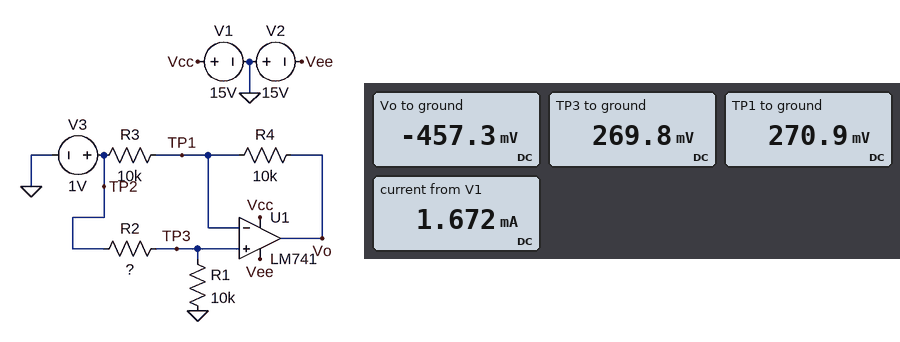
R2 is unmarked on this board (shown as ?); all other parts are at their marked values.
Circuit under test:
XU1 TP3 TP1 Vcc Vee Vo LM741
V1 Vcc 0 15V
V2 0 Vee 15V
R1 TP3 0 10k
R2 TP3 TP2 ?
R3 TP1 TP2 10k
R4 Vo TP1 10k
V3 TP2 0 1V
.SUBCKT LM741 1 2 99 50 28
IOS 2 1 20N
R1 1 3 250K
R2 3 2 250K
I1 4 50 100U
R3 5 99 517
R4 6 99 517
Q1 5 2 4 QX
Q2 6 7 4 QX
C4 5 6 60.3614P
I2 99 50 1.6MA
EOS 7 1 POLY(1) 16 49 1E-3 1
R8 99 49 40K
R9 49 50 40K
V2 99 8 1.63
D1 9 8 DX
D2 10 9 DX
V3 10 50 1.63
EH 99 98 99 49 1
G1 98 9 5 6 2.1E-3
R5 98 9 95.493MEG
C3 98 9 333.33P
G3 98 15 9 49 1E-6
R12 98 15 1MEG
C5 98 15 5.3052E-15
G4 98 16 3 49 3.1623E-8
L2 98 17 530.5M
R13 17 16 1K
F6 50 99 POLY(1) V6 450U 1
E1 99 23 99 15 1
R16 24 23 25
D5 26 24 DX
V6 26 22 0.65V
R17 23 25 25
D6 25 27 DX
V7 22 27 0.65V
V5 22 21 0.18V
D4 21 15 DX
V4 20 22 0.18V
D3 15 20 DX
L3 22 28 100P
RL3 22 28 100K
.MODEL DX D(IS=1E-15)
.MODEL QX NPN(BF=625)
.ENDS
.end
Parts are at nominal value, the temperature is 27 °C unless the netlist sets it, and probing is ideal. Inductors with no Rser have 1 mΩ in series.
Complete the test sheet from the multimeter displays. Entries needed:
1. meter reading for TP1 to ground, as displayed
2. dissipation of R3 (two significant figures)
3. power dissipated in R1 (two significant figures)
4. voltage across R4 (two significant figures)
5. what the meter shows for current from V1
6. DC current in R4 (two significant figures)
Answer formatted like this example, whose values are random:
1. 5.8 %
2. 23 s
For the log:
1. 270.9 mV
2. 53 µW
3. 7.3 µW
4. 730 mV
5. 1.672 mA
6. 73 µA
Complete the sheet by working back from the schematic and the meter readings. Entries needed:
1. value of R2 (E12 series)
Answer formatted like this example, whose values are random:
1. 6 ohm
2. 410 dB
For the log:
1. 27 kΩ
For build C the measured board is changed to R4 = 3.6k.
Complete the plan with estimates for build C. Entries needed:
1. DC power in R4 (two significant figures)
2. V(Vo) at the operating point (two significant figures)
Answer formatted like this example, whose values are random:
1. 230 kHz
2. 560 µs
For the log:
1. 19 µW
2. 8.7 mV
